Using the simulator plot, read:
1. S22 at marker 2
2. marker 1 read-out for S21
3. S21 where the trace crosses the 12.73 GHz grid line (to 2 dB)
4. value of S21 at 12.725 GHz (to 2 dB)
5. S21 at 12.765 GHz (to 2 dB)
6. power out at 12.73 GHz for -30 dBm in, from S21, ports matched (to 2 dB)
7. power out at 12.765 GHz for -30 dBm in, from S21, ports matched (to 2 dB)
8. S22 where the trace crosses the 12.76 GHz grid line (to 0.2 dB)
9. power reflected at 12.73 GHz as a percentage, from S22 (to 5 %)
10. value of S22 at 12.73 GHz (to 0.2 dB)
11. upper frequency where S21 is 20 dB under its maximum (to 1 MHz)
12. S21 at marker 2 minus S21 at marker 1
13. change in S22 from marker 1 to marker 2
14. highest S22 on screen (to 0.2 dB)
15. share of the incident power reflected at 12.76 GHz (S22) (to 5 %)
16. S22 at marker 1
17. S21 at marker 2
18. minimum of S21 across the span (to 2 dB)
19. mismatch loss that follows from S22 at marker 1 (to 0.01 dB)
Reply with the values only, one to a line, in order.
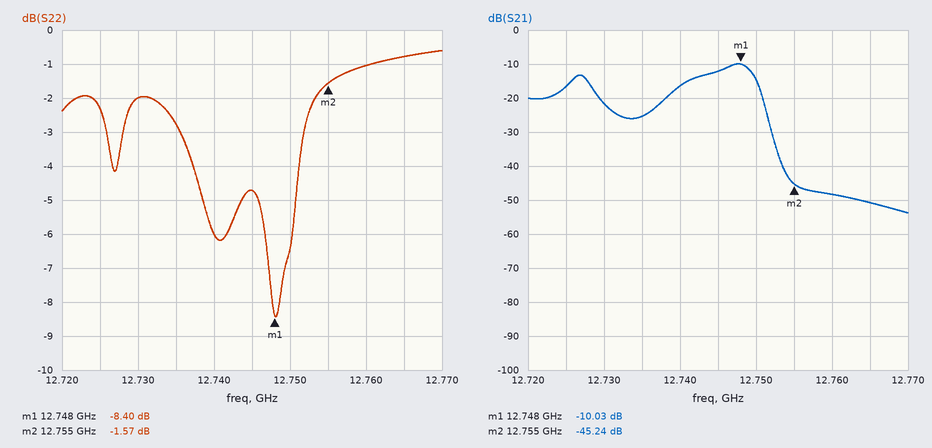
-1.57 dB
-10.03 dB
-22 dB
-16 dB
-50 dB
-52 dBm
-80 dBm
-1.0 dB
65 %
-2.0 dB
12.752 GHz
-35.21 dB
6.83 dB
-0.6 dB
80 %
-8.40 dB
-45.24 dB
-54 dB
0.68 dB
